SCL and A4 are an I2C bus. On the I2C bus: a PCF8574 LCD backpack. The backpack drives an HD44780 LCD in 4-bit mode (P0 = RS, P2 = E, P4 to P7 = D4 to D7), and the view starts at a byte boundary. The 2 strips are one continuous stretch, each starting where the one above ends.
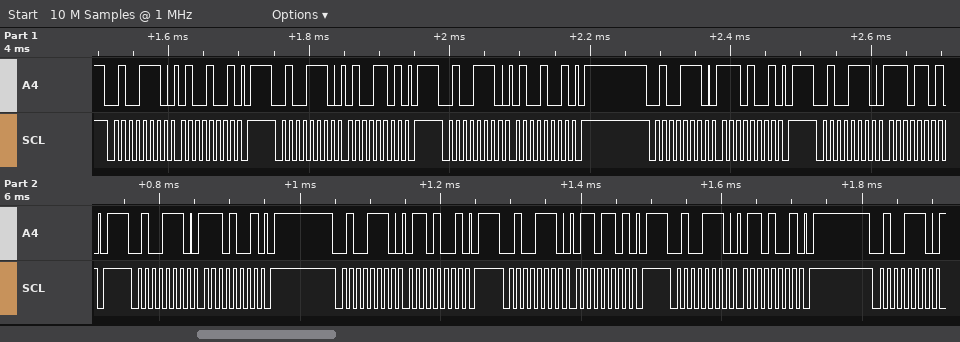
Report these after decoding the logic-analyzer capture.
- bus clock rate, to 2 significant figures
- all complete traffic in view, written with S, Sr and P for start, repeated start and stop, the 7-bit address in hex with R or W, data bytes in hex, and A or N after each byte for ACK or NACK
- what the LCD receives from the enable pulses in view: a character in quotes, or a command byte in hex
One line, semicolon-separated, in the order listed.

100 kHz; S 27W A 49 A P S 27W A 4D A P S 27W A 49 A P S 27W A E9 A P S 27W A ED A P S 27W A E9 A P S 27W A 69 A P S 27W A 6D A P S 27W A 69 A P S 27W A; 'N'
